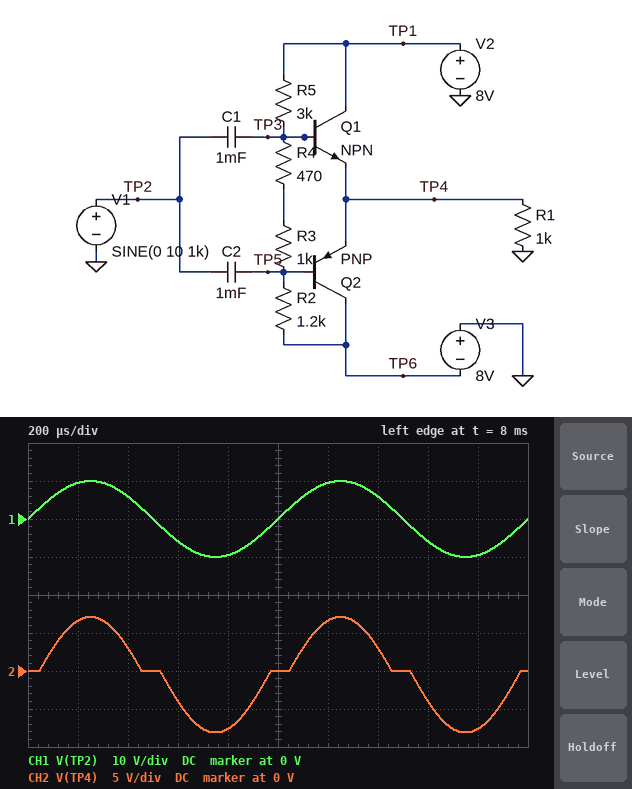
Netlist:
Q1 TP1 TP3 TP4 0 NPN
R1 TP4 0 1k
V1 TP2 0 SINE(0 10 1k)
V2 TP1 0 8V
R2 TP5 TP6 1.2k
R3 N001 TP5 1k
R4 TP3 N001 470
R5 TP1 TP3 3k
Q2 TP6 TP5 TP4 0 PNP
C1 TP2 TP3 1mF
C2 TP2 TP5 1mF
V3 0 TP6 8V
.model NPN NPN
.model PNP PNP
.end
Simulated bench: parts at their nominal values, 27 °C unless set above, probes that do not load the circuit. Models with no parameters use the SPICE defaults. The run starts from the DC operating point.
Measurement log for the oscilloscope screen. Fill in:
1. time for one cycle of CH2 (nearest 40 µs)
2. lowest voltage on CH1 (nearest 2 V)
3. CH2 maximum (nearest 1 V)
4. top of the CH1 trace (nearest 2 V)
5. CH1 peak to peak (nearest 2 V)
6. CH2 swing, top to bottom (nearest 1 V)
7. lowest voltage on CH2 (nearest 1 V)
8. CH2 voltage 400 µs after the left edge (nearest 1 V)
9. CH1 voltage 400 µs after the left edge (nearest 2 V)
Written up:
1.00 ms
-10 V
7 V
10 V
20 V
15 V
-8 V
3 V
6 V
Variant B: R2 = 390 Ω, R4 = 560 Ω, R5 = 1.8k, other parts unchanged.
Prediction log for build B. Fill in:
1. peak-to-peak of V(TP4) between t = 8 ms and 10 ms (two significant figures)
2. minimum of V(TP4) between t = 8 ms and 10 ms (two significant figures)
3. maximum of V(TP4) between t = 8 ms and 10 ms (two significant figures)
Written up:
14 V
-8.0 V
5.7 V
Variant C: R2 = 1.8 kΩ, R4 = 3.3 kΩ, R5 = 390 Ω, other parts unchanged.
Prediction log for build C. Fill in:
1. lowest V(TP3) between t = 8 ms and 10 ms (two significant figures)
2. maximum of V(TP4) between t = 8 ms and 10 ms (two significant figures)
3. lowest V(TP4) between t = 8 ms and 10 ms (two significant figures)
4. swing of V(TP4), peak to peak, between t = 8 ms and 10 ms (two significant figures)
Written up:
-11 V
8.0 V
-5.7 V
14 V
